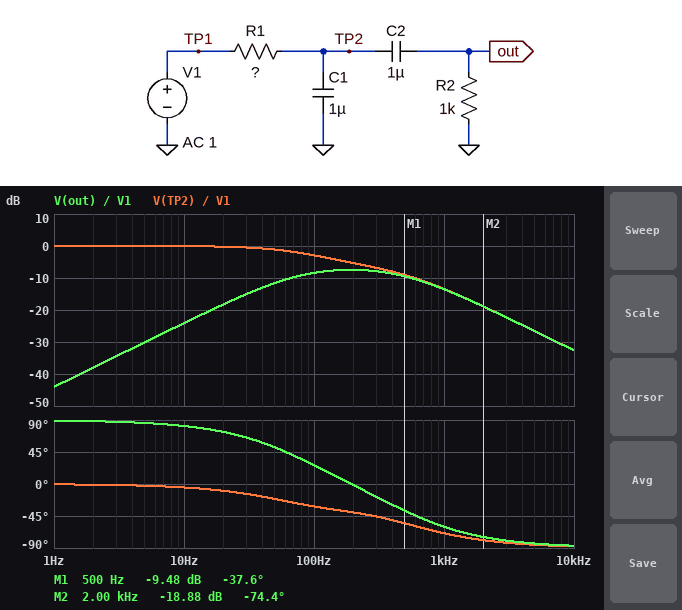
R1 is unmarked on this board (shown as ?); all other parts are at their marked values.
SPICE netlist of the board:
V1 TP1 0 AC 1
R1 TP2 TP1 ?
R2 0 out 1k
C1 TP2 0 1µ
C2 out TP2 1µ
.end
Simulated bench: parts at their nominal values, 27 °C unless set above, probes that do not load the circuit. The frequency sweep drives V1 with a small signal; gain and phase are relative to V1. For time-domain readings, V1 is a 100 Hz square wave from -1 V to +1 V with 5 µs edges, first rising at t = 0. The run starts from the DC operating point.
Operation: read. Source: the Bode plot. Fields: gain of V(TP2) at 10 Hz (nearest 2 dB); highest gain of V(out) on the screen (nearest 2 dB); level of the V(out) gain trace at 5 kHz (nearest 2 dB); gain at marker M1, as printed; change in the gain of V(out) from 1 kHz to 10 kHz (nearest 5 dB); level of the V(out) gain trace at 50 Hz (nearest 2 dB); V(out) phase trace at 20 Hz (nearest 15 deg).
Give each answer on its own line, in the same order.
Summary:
0 dB
-8 dB
-26 dB
-9.48 dB
-20 dB
-12 dB
75 deg
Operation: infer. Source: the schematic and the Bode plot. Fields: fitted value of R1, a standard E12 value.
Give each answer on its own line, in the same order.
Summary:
680 Ω
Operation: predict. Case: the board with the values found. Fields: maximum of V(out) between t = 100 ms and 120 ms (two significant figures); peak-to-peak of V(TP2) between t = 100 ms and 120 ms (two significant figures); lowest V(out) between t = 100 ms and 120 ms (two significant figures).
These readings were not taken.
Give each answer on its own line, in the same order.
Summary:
630 mV
1.8 V
-630 mV
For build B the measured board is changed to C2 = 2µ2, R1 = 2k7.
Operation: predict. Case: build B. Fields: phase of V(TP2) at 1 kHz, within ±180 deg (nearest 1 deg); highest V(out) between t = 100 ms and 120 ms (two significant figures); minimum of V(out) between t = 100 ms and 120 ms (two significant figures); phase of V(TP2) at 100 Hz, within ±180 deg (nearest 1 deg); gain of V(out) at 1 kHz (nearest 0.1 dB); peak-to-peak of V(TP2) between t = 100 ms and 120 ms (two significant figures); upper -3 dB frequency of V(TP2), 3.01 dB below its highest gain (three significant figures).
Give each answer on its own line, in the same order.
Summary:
-78 deg
220 mV
-220 mV
-47 deg
-24.9 dB
730 mV
16.2 Hz
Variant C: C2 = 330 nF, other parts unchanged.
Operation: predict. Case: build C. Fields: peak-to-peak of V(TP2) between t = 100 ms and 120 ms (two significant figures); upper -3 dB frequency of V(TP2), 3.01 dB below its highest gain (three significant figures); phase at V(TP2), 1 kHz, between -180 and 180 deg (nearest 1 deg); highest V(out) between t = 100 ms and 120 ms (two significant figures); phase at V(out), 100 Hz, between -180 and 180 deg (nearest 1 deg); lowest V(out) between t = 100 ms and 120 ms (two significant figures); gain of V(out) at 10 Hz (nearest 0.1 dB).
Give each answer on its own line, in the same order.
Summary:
2.0 V
167 Hz
-71 deg
420 mV
50 deg
-420 mV
-33.7 dB
